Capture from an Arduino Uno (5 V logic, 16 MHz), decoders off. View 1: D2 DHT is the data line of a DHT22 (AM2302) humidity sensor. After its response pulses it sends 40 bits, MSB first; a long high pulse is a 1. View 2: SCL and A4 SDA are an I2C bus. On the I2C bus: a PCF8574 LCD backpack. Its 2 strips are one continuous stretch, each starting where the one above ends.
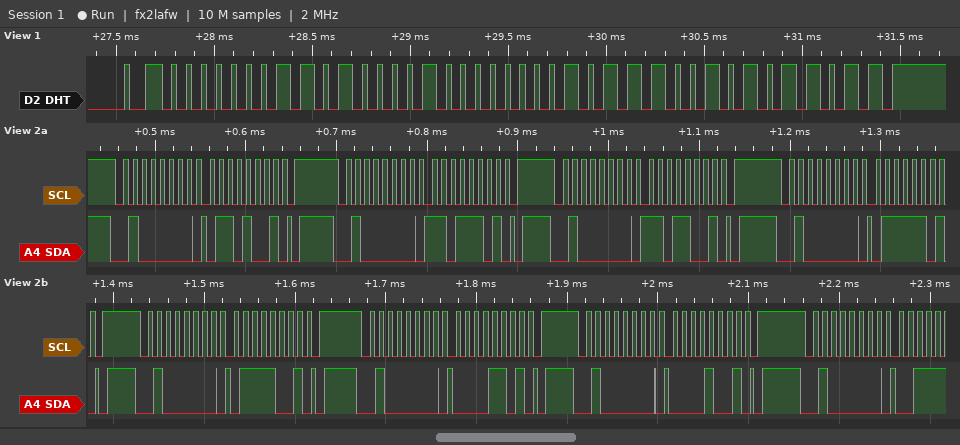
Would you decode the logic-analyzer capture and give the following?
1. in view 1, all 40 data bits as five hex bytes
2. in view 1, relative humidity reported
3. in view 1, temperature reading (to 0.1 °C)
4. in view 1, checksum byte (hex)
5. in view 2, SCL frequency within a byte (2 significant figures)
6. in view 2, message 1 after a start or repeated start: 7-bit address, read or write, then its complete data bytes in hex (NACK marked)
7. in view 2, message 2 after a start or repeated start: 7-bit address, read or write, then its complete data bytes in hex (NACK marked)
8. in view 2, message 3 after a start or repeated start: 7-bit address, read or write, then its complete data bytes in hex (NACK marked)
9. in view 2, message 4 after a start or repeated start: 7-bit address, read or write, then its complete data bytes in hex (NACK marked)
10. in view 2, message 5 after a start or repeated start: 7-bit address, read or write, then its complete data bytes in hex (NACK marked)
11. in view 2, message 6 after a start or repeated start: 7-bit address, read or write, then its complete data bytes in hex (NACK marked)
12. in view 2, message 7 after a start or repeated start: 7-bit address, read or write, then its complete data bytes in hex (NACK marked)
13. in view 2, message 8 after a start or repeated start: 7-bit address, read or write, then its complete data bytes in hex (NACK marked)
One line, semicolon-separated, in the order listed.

01 A1 00 B9 5B; 41.7 %; 18.5 °C; 0x5B; 100 kHz; 0x20 write: 69; 0x20 write: DD; 0x20 write: D9; 0x20 write: 7D; 0x20 write: 79; 0x20 write: 0D; 0x20 write: 09; 0x20 write
